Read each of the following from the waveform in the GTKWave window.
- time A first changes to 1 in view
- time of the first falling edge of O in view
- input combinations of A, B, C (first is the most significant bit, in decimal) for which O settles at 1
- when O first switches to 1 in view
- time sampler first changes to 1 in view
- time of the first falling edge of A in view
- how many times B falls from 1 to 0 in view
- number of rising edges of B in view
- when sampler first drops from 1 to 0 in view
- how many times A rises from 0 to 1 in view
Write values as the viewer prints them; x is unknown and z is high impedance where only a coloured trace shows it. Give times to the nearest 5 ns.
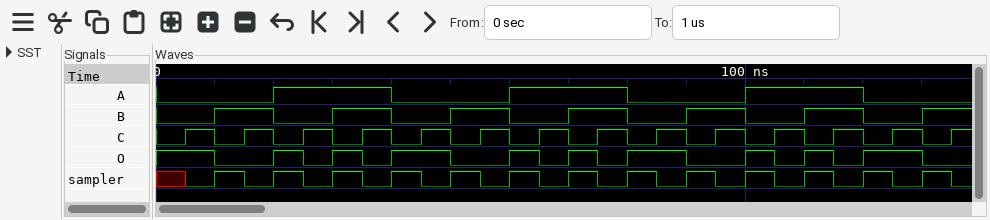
20 ns
10 ns
0, 1, 4, 6
20 ns
10 ns
40 ns
6
7
15 ns
3
